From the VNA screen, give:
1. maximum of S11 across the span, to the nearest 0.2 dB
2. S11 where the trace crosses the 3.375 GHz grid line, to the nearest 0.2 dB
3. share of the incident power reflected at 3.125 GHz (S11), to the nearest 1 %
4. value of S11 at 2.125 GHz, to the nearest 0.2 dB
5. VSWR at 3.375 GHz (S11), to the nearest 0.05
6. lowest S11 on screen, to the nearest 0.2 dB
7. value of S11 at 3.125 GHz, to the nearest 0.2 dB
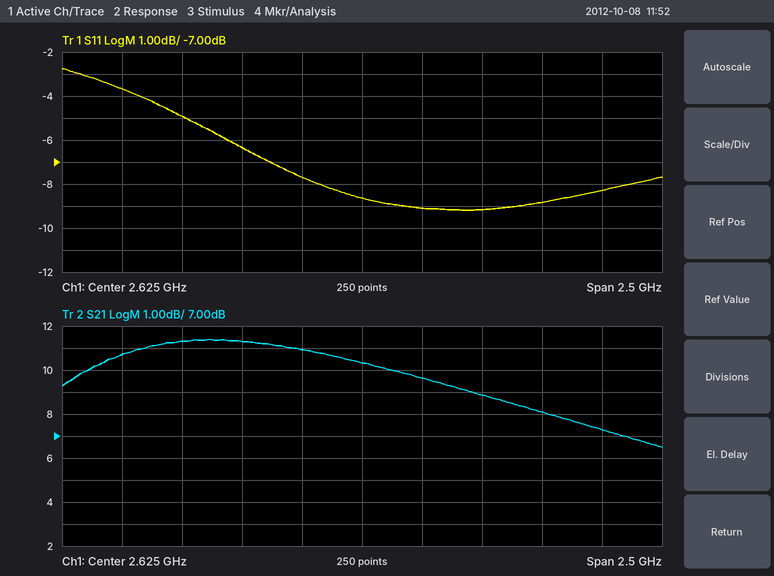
-2.8 dB
-8.8 dB
12 %
-6.4 dB
2.15
-9.2 dB
-9.2 dB
